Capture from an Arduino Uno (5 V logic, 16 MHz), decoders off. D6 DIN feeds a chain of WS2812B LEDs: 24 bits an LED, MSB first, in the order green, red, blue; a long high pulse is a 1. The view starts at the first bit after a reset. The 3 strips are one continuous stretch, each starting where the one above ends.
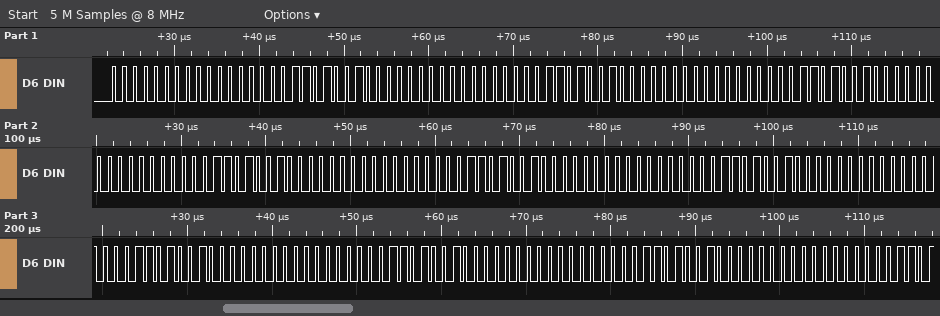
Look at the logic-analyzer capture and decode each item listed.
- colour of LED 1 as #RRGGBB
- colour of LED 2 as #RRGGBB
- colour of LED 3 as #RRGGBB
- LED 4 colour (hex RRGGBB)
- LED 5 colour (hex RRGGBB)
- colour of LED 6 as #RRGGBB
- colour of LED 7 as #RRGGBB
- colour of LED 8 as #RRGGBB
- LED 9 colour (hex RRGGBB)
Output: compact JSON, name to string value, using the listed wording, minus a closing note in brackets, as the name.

{"colour of LED 1 as #RRGGBB": "#000069", "colour of LED 2 as #RRGGBB": "#000069", "colour of LED 3 as #RRGGBB": "#000069", "LED 4 colour": "#000069", "LED 5 colour": "#000069", "colour of LED 6 as #RRGGBB": "#000069", "colour of LED 7 as #RRGGBB": "#000069", "colour of LED 8 as #RRGGBB": "#000069", "LED 9 colour": "#000069"}
